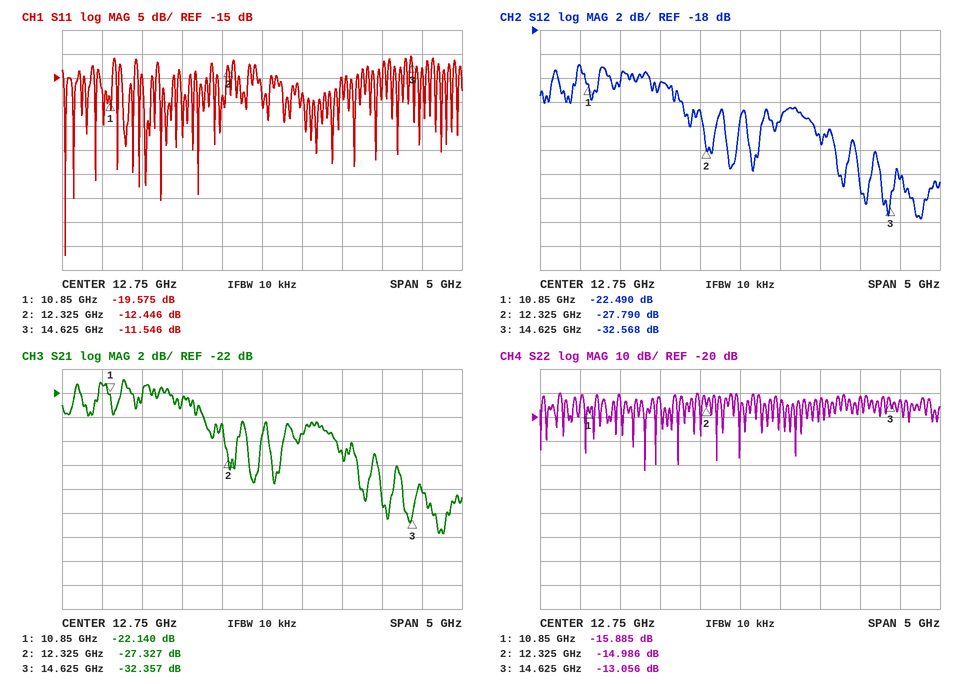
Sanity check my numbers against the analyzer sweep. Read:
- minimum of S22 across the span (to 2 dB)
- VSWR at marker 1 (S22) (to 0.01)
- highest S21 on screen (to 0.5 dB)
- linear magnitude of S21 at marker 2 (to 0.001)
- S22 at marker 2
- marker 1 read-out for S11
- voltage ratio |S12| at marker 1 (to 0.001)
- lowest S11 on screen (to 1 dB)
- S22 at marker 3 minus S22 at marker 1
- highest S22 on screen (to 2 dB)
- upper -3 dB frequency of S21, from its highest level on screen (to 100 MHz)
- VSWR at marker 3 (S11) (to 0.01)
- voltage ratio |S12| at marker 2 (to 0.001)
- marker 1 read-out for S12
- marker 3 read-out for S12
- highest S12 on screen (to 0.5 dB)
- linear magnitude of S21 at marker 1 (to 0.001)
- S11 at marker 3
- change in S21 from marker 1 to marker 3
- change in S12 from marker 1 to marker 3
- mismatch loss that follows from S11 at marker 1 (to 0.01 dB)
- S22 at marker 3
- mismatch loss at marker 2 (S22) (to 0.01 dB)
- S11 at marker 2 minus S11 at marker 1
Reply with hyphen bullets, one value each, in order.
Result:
- -42 dB
- 1.38
- -21.0 dB
- 0.043
- -14.986 dB
- -19.575 dB
- 0.075
- -52 dB
- 2.829 dB
- -10 dB
- 12.0 GHz
- 1.72
- 0.041
- -22.490 dB
- -32.568 dB
- -21.0 dB
- 0.078
- -11.546 dB
- -10.217 dB
- -10.078 dB
- 0.05 dB
- -13.056 dB
- 0.14 dB
- 7.129 dB
